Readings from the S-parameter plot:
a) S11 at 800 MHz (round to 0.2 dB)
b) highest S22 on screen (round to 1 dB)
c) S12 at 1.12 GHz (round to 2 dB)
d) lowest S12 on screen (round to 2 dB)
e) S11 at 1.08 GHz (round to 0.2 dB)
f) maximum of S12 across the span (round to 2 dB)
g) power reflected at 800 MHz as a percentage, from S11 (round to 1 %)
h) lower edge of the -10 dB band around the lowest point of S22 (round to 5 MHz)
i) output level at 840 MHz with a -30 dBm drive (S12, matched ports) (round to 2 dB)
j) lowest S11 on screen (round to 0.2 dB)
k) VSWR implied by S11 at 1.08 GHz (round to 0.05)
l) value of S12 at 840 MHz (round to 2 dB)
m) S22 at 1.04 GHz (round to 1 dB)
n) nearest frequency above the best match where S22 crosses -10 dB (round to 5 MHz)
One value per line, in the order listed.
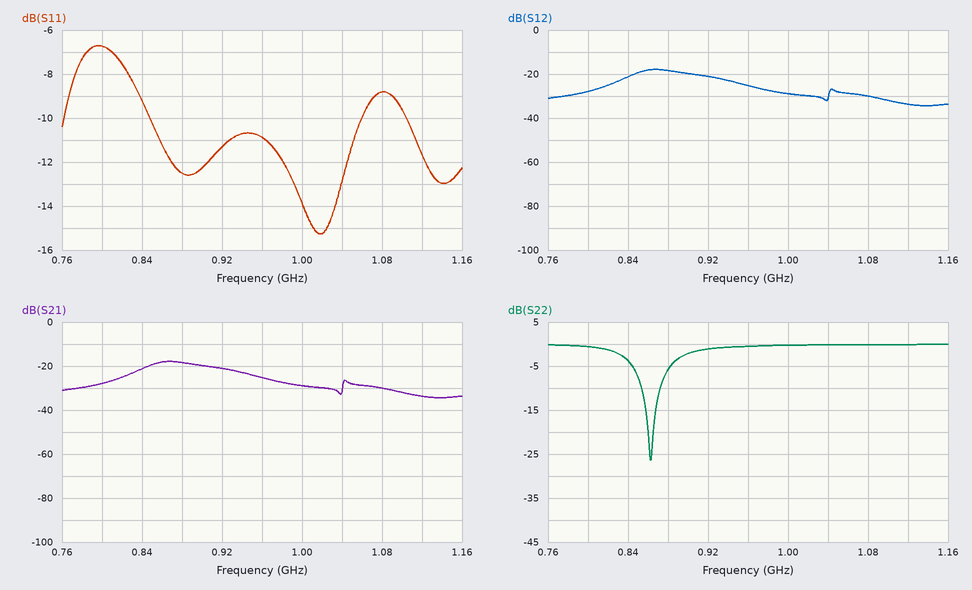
-6.8 dB
0 dB
-34 dB
-34 dB
-8.8 dB
-18 dB
21 %
855 MHz
-52 dBm
-15.2 dB
2.15
-22 dB
0 dB
870 MHz
